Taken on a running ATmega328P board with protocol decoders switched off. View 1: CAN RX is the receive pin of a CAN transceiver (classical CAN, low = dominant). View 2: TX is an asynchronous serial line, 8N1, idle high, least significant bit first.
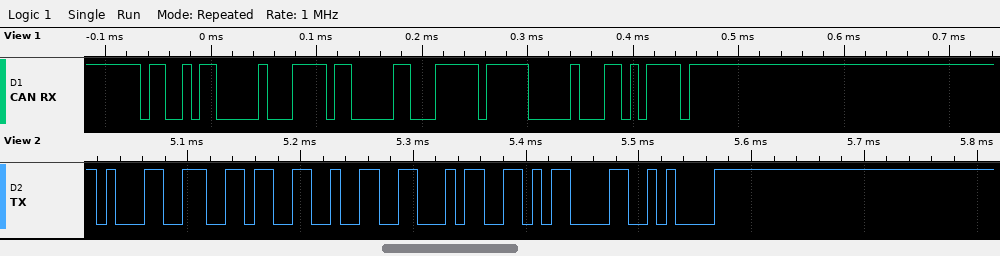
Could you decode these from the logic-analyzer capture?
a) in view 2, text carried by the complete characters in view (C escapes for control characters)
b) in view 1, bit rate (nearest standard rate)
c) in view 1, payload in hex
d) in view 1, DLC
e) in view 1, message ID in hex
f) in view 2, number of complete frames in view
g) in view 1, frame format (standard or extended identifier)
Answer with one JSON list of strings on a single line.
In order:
["\"1624\\r\\n\"", "125 kbit/s", "D8 23 FF", "3", "0x658", "6", "standard"]
